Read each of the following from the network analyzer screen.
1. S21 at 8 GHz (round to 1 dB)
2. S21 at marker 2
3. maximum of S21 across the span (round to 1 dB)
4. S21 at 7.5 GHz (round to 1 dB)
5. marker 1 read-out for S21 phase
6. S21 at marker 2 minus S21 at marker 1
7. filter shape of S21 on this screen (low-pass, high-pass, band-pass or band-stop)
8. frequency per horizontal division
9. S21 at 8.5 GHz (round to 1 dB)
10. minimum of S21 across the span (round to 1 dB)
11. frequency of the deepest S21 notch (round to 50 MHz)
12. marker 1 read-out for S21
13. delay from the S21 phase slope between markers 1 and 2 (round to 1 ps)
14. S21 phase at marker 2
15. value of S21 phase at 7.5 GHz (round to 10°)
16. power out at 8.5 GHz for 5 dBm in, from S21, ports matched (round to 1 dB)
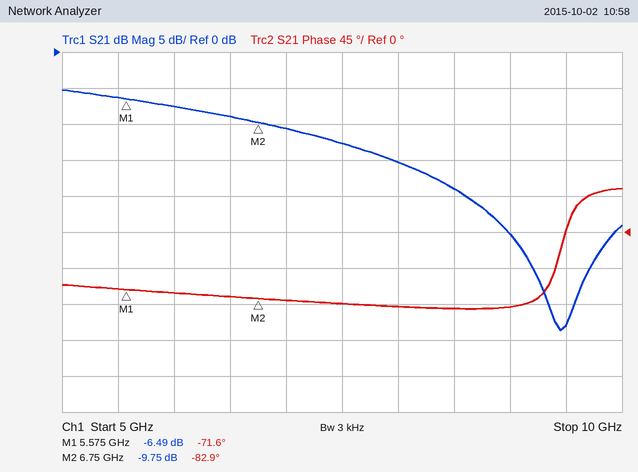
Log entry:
-15 dB
-9.75 dB
-5 dB
-13 dB
-71.6°
-3.26 dB
low-pass
500 MHz
-19 dB
-39 dB
9.45 GHz
-6.49 dB
27 ps
-82.9°
-90°
-14 dBm
